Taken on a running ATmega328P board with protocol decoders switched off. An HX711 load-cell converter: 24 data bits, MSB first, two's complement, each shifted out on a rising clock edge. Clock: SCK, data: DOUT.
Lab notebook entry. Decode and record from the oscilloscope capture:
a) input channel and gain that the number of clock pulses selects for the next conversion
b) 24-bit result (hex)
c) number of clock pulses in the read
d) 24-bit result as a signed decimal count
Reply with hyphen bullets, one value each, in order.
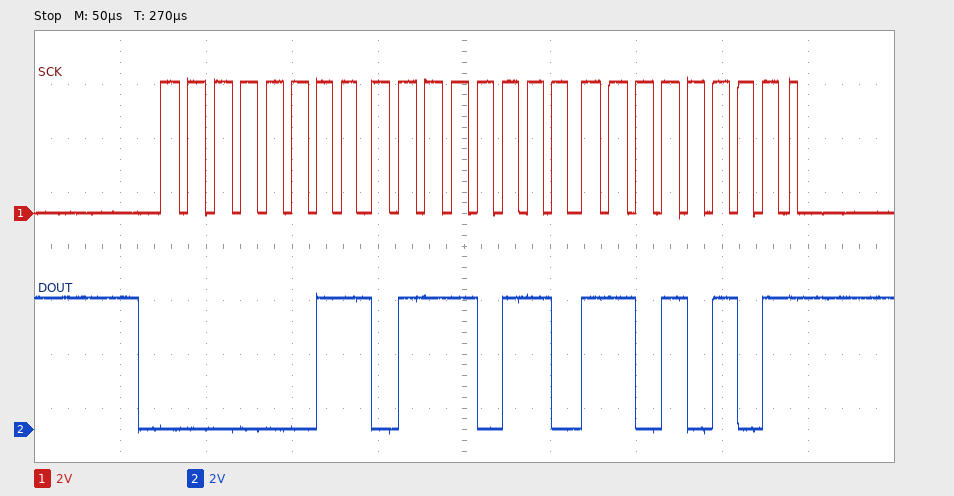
- channel A, gain 128
- 0x0376D5
- 25
- 227029
